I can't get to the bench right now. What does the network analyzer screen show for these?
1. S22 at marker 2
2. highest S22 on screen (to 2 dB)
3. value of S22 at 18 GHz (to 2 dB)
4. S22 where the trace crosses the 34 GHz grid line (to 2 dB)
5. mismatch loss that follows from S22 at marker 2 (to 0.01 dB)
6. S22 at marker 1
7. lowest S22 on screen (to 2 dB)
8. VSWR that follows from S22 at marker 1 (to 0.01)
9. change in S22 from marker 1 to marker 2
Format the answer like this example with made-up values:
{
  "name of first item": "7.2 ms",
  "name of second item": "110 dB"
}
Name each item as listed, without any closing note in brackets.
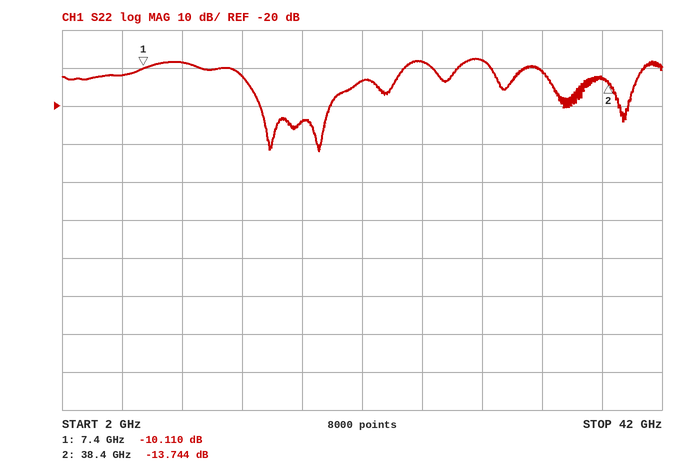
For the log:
{
  "S22 at marker 2": "-13.744 dB",
  "highest S22 on screen": "-8 dB",
  "value of S22 at 18 GHz": "-24 dB",
  "S22 where the trace crosses the 34 GHz grid line": "-10 dB",
  "mismatch loss that follows from S22 at marker 2": "0.19 dB",
  "S22 at marker 1": "-10.110 dB",
  "lowest S22 on screen": "-32 dB",
  "VSWR that follows from S22 at marker 1": "1.91",
  "change in S22 from marker 1 to marker 2": "-3.634 dB"
}
